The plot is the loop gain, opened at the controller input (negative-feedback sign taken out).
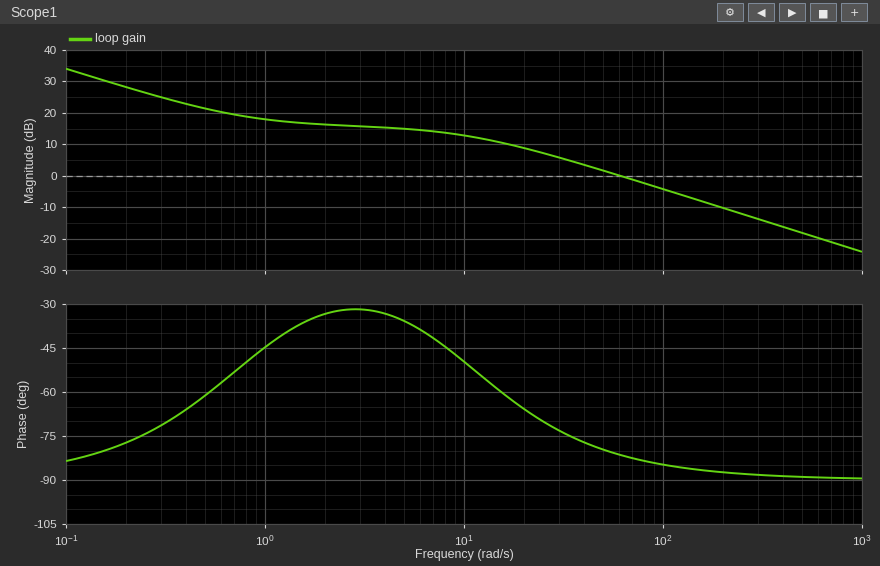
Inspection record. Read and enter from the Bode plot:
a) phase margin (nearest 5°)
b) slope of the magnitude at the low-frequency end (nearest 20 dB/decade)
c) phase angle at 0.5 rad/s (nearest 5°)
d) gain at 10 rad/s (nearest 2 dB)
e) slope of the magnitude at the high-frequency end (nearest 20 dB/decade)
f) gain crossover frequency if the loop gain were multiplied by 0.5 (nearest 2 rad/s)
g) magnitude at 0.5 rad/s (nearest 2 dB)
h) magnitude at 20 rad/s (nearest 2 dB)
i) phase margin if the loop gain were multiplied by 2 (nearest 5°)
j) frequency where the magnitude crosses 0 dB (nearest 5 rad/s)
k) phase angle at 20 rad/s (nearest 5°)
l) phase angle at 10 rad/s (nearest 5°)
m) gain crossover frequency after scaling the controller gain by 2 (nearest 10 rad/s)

100°
-20 dB/decade
-60°
12 dB
-20 dB/decade
30 rad/s
22 dB
8 dB
95°
60 rad/s
-65°
-50°
120 rad/s
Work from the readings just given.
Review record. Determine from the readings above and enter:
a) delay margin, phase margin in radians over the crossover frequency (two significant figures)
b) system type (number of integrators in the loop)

0.029 s
1
